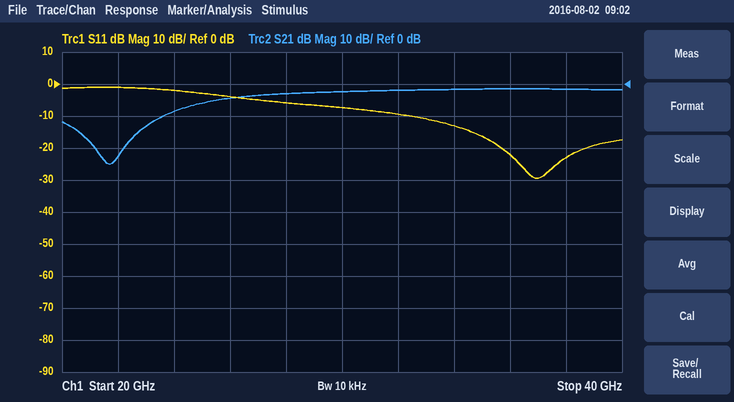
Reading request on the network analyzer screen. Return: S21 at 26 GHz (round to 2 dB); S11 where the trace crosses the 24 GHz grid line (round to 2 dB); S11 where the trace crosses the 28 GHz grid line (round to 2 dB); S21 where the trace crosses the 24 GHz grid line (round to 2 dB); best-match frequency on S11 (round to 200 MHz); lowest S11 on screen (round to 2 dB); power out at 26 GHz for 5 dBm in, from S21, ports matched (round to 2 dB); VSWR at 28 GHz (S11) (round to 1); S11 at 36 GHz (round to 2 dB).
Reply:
-4 dB
-2 dB
-6 dB
-8 dB
37.0 GHz
-30 dB
0 dBm
3
-22 dB
